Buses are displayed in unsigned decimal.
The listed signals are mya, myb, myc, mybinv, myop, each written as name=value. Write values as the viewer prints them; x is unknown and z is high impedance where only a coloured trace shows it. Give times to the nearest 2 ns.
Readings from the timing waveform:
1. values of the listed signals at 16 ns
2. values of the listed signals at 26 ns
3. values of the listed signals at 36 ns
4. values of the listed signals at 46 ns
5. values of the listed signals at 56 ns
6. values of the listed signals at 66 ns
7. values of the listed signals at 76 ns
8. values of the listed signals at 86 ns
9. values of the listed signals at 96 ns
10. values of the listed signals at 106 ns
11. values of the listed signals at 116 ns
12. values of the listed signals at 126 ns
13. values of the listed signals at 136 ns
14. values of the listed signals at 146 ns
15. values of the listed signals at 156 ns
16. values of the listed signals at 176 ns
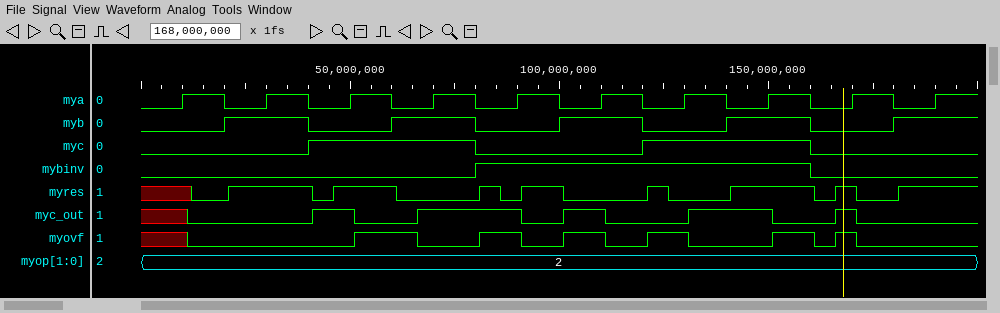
mya=1, myb=0, myc=0, mybinv=0, myop=2
mya=0, myb=1, myc=0, mybinv=0, myop=2
mya=1, myb=1, myc=0, mybinv=0, myop=2
mya=0, myb=0, myc=1, mybinv=0, myop=2
mya=1, myb=0, myc=1, mybinv=0, myop=2
mya=0, myb=1, myc=1, mybinv=0, myop=2
mya=1, myb=1, myc=1, mybinv=0, myop=2
mya=0, myb=0, myc=0, mybinv=1, myop=2
mya=1, myb=0, myc=0, mybinv=1, myop=2
mya=0, myb=1, myc=0, mybinv=1, myop=2
mya=1, myb=1, myc=0, mybinv=1, myop=2
mya=0, myb=0, myc=1, mybinv=1, myop=2
mya=1, myb=0, myc=1, mybinv=1, myop=2
mya=0, myb=1, myc=1, mybinv=1, myop=2
mya=1, myb=1, myc=1, mybinv=1, myop=2
mya=1, myb=0, myc=0, mybinv=0, myop=2
